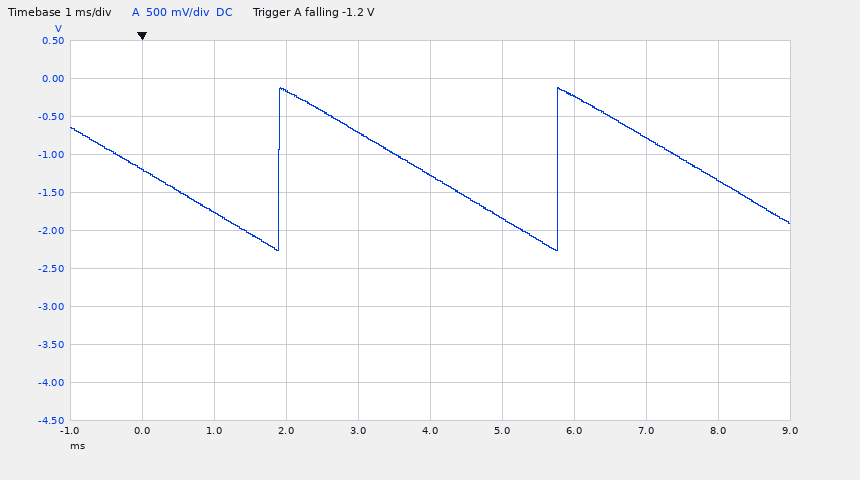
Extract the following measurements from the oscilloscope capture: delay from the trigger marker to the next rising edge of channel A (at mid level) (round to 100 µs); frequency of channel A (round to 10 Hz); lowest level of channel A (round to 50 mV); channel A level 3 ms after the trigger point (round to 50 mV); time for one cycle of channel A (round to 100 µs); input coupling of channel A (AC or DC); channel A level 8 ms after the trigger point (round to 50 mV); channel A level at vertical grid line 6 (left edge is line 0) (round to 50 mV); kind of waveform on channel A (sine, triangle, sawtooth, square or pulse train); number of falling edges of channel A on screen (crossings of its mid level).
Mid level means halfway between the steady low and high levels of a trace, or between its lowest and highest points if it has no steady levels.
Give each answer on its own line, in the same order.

1.9 ms
260 Hz
-2.25 V
-700 mV
3.9 ms
DC
-1.35 V
-1.85 V
sawtooth
3
